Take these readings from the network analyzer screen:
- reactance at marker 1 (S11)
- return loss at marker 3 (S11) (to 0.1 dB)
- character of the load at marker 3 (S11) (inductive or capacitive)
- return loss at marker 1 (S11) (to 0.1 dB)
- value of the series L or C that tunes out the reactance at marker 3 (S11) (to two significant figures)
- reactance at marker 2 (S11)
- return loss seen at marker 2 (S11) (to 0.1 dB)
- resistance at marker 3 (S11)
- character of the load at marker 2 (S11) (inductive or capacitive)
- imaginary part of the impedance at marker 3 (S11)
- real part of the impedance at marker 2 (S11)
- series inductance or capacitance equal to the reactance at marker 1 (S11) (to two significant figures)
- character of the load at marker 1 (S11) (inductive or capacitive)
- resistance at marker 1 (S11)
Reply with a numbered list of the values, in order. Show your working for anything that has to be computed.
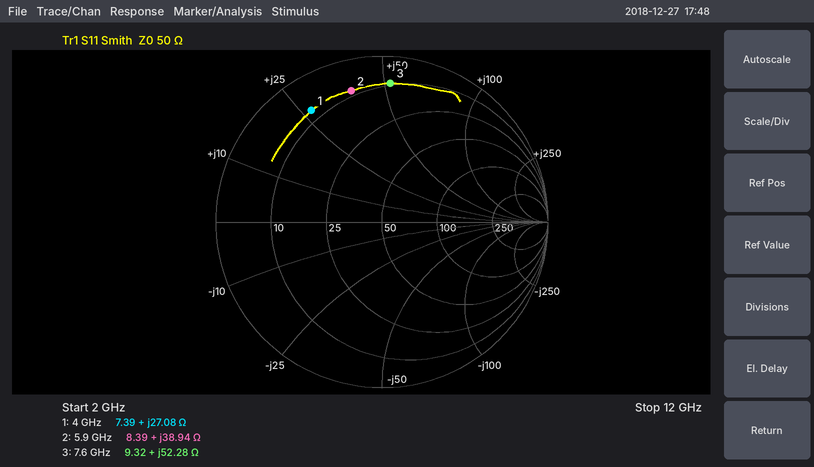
1. +27.08 Ω
2. 1.5 dB
3. inductive
4. 2.0 dB
5. C = 1/(2π × 7.6 GHz × 52.28 Ω) ≈ 401 fF, so 400 fF to two significant figures
6. +38.94 Ω
7. 1.8 dB
8. 9.32 Ω
9. inductive
10. +52.28 Ω
11. 8.39 Ω
12. L = 27.08 Ω/(2π × 4 GHz) ≈ 1.1 nH
13. inductive
14. 7.39 Ω
